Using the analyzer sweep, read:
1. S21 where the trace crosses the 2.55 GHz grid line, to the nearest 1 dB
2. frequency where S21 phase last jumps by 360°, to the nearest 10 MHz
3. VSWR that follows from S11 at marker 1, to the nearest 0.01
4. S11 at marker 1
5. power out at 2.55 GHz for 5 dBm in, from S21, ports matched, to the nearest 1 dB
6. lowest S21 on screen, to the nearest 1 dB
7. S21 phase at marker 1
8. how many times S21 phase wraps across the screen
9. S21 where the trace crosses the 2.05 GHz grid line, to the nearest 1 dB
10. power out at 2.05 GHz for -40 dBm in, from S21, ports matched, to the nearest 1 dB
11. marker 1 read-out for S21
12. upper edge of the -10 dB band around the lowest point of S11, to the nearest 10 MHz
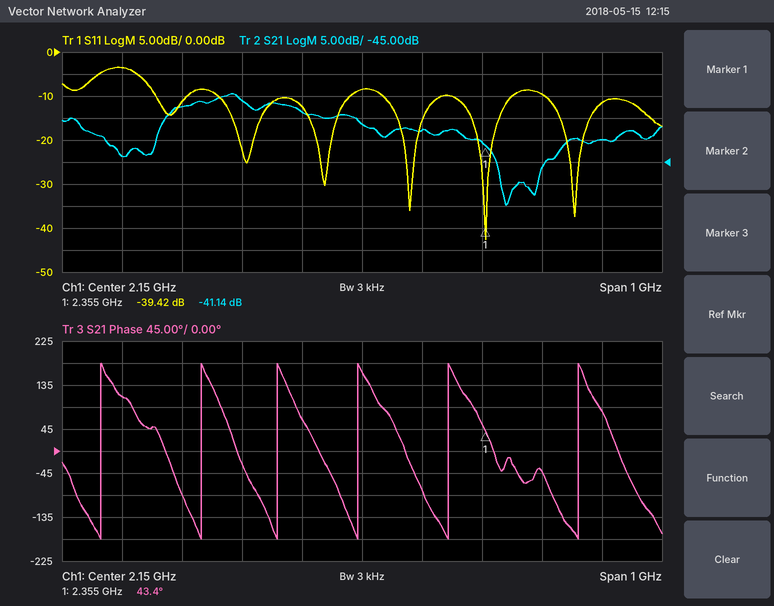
-40 dB
2.51 GHz
1.02
-39.42 dB
-35 dBm
-55 dB
43.4°
6
-34 dB
-74 dBm
-41.14 dB
2.40 GHz
